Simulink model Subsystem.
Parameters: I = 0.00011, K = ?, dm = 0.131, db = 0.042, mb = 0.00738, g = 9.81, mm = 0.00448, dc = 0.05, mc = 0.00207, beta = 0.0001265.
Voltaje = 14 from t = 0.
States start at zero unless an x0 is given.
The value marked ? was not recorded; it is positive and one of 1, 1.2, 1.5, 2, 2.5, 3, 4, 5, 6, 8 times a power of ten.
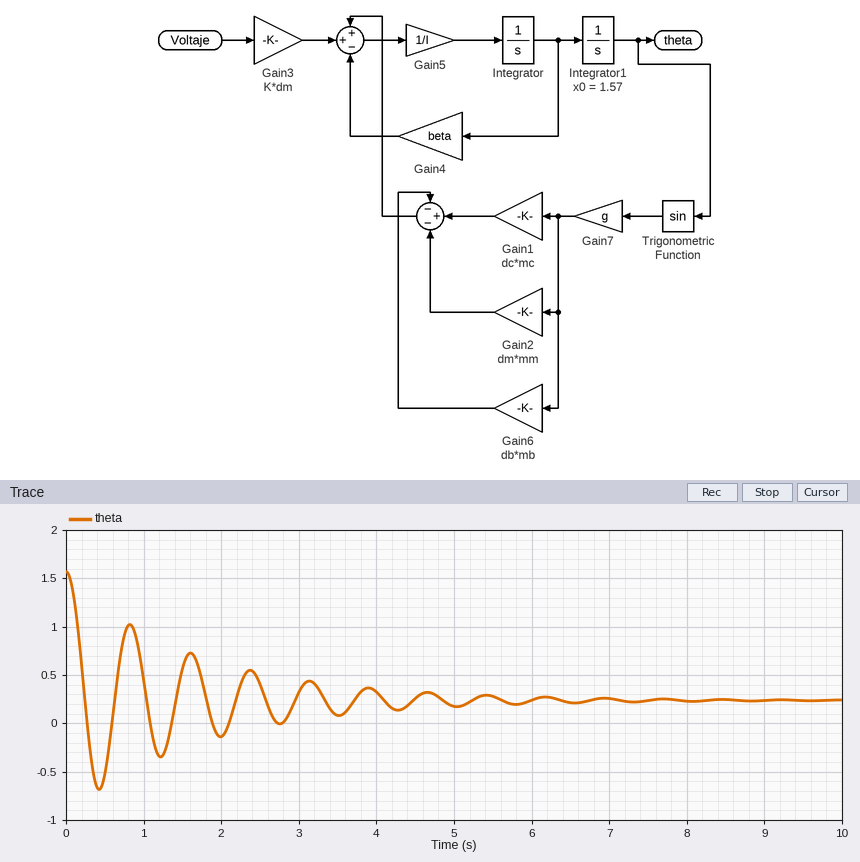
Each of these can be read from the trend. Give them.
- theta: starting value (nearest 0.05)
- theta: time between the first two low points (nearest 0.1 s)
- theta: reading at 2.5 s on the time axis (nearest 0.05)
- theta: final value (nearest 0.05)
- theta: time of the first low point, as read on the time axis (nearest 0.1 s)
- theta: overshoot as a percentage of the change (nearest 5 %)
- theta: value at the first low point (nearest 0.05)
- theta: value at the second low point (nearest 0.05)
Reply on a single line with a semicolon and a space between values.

1.55; 0.8 s; 0.40; 0.25; 0.4 s; 70 %; -0.70; -0.35
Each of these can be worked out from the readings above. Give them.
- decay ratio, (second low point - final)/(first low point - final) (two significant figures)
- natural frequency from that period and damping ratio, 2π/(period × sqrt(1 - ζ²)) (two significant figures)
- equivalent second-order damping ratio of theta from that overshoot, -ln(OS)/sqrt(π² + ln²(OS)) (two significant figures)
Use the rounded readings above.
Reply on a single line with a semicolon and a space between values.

0.63; 7.9 rad/s; 0.11
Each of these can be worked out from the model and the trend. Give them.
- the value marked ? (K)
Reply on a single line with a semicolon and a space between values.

0.001
